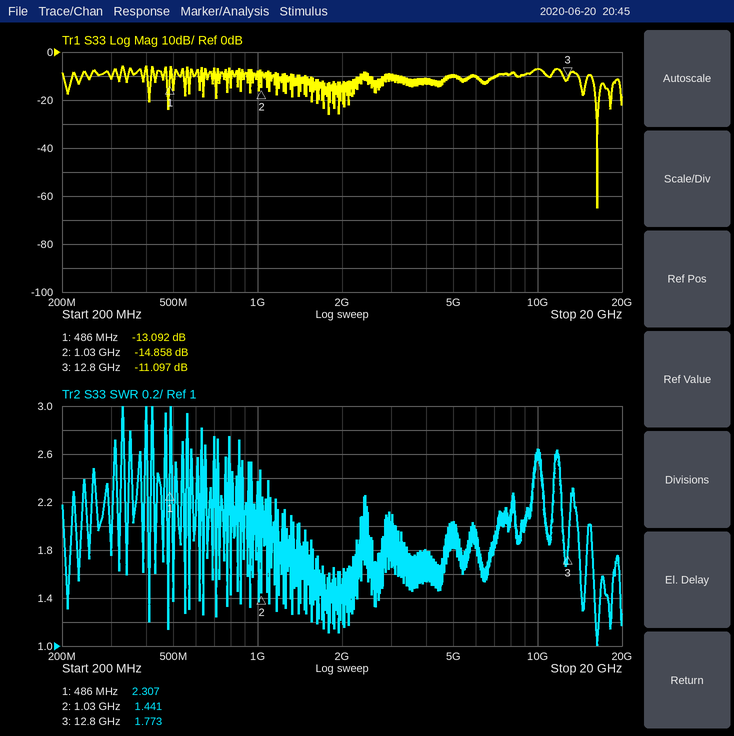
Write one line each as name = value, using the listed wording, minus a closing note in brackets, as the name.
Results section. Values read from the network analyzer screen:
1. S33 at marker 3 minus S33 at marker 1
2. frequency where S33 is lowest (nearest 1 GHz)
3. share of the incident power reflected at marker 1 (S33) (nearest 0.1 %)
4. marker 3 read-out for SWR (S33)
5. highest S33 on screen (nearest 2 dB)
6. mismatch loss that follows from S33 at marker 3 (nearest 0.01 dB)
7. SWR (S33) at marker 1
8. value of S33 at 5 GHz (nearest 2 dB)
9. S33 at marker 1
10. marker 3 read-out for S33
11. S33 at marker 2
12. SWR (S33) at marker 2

S33 at marker 3 minus S33 at marker 1 = 1.995 dB
frequency where S33 is lowest = 16 GHz
share of the incident power reflected at marker 1 (S33) = 4.9 %
marker 3 read-out for SWR = 1.773
highest S33 on screen = -6 dB
mismatch loss that follows from S33 at marker 3 = 0.35 dB
SWR (S33) at marker 1 = 2.307
value of S33 at 5 GHz = -10 dB
S33 at marker 1 = -13.092 dB
marker 3 read-out for S33 = -11.097 dB
S33 at marker 2 = -14.858 dB
SWR (S33) at marker 2 = 1.441
